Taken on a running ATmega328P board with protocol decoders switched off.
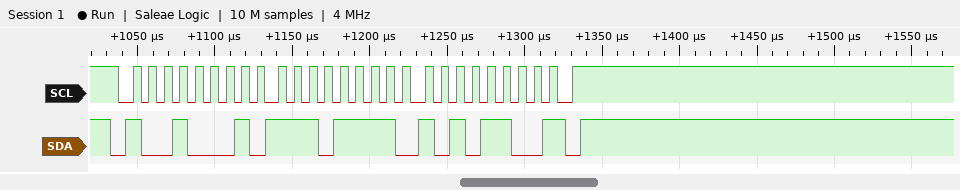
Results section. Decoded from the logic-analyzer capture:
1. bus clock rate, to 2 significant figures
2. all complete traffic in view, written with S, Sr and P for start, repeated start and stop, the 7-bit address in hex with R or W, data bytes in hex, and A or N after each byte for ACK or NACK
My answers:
100 kHz
S 48R A EF A AC N P
